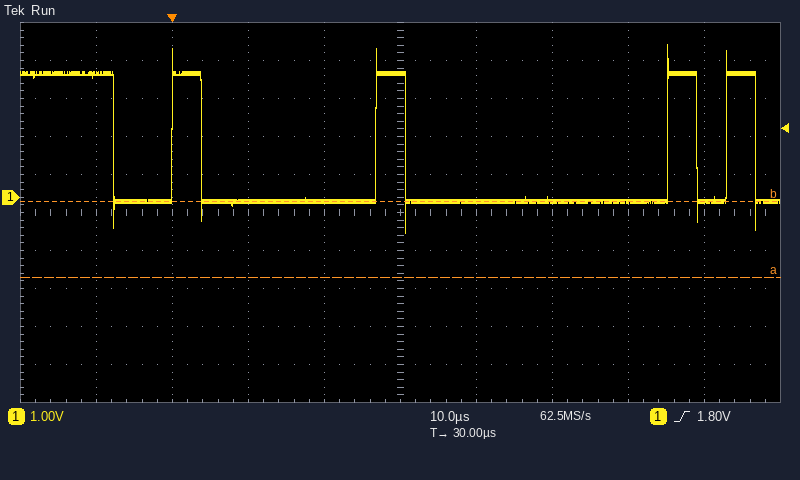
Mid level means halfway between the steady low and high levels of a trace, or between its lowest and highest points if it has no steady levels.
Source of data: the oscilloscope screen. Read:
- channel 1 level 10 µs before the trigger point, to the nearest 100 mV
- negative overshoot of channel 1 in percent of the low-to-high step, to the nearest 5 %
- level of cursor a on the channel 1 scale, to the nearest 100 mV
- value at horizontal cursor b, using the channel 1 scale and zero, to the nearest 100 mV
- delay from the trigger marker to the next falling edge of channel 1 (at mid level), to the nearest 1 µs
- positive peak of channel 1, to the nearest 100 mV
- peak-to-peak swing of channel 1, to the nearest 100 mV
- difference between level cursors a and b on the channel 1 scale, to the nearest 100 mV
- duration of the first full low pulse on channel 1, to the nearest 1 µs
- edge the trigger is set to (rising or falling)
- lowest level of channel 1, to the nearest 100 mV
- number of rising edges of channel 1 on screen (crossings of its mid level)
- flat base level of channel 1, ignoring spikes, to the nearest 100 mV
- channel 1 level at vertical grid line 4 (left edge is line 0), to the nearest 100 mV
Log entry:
3.2 V
25 %
-2.1 V
-100 mV
4 µs
4.0 V
4.9 V
2.0 V
8 µs
rising
-900 mV
4
-100 mV
-100 mV
